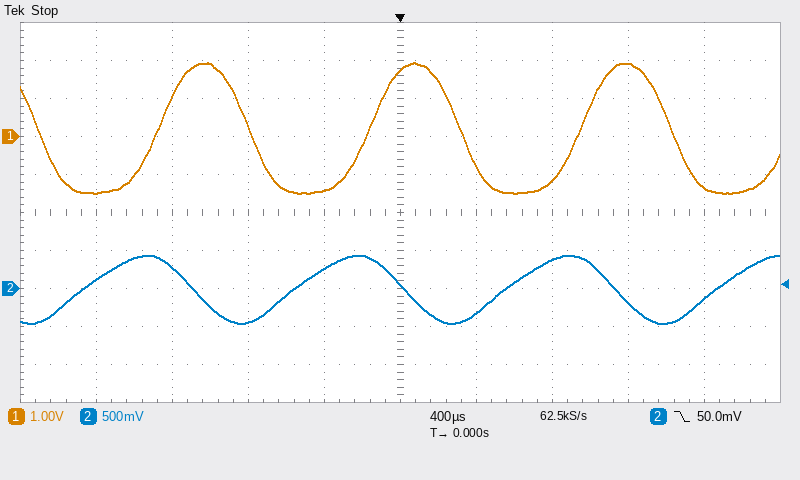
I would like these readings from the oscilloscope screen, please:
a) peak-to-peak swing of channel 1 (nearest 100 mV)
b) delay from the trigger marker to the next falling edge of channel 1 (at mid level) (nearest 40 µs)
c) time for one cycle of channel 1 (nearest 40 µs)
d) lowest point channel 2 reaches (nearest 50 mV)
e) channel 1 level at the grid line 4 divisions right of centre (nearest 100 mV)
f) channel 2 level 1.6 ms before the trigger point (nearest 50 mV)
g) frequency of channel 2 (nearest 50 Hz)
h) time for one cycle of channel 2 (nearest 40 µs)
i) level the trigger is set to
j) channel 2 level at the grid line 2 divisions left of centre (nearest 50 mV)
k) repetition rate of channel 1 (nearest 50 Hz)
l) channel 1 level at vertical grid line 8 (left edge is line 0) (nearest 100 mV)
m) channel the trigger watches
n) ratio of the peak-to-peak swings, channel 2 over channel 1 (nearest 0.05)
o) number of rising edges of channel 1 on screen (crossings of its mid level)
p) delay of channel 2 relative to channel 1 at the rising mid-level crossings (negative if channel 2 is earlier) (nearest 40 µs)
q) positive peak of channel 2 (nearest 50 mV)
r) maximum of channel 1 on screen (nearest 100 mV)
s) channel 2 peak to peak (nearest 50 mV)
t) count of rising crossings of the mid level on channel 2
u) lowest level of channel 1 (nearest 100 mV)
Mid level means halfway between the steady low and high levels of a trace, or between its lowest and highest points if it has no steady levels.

3.4 V
320 µs
1.12 ms
-450 mV
-1.3 V
100 mV
900 Hz
1.12 ms
50.0 mV
-450 mV
900 Hz
1.9 V
channel 2
0.25
3
-400 µs
450 mV
1.9 V
900 mV
4
-1.5 V
